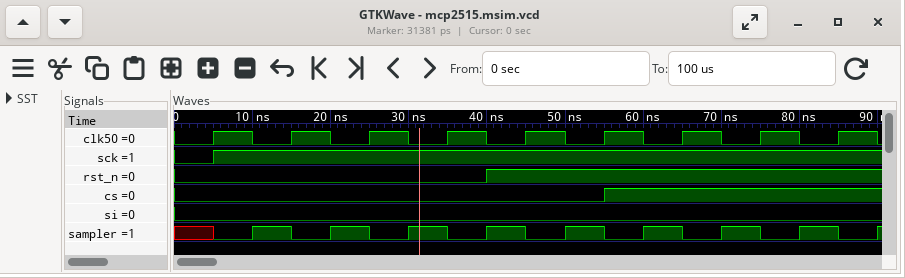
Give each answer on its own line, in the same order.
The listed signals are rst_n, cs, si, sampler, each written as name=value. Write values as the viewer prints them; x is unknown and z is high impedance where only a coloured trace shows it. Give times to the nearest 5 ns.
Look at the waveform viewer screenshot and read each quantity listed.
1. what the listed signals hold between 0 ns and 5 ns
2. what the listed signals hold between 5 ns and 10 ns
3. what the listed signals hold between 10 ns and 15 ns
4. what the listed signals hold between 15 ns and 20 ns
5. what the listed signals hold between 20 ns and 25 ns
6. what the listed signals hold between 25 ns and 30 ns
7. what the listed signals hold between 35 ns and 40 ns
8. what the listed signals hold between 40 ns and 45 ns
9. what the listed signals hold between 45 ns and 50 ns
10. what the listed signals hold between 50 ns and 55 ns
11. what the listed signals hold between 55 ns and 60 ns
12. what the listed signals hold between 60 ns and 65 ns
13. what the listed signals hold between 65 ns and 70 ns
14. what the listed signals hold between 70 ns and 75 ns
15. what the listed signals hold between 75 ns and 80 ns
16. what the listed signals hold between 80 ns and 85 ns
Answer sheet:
rst_n=0, cs=0, si=0, sampler=x
rst_n=0, cs=0, si=0, sampler=0
rst_n=0, cs=0, si=0, sampler=1
rst_n=0, cs=0, si=0, sampler=0
rst_n=0, cs=0, si=0, sampler=1
rst_n=0, cs=0, si=0, sampler=0
rst_n=0, cs=0, si=0, sampler=0
rst_n=1, cs=0, si=0, sampler=1
rst_n=1, cs=0, si=0, sampler=0
rst_n=1, cs=0, si=0, sampler=1
rst_n=1, cs=1, si=0, sampler=0
rst_n=1, cs=1, si=0, sampler=1
rst_n=1, cs=1, si=0, sampler=0
rst_n=1, cs=1, si=0, sampler=1
rst_n=1, cs=1, si=0, sampler=0
rst_n=1, cs=1, si=0, sampler=1
